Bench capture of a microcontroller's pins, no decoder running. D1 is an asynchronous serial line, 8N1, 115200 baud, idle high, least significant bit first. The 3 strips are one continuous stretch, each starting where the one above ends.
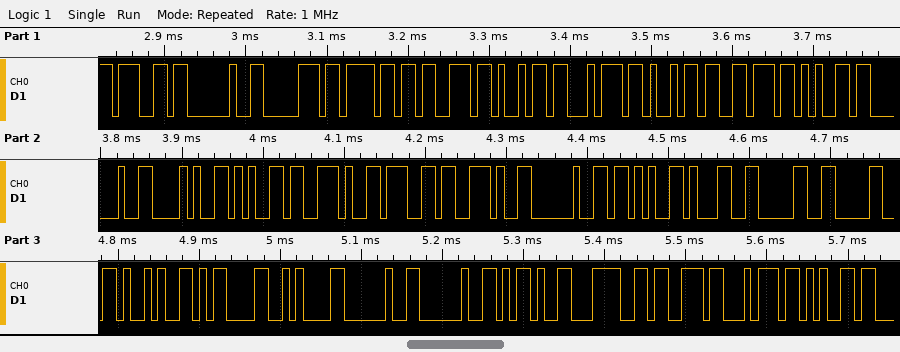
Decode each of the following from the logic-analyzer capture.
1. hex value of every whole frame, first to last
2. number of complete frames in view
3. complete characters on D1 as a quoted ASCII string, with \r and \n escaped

0x67 0x20 0x70 0x6F 0x73 0x69 0x74 0x69 0x76 0x65 0x20 0x28 0x65 0x2E 0x67 0x2E 0x20 0x2B 0x31 0x30 0x30 0x29 0x0D 0x0A 0x20 0x20 0x2D 0x3C 0x73 0x74 0x65
31
"g positive (e.g. +100)\r\n  -<ste"
